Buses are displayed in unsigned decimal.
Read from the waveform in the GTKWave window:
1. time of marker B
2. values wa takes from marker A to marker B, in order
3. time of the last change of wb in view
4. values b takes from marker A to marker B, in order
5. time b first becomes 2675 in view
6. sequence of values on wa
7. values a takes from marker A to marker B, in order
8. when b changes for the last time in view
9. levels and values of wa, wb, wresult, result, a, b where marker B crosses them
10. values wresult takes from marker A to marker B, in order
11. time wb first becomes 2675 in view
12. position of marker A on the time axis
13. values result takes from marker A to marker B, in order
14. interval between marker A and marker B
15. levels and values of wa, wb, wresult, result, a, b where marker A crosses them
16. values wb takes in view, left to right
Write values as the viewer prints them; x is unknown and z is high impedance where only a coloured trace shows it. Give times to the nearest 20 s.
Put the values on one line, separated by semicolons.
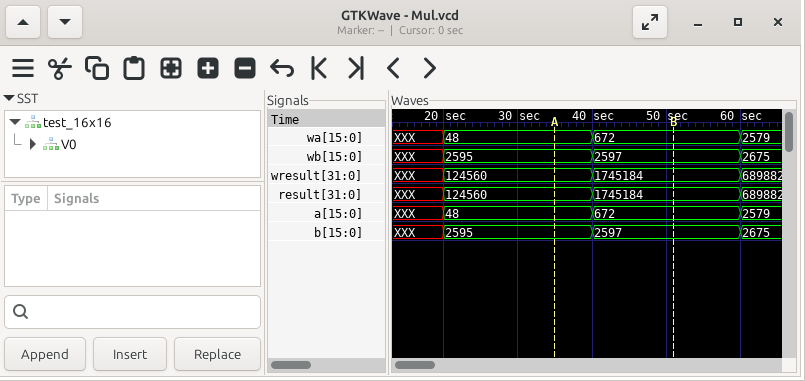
60 s; 48, 672; 60 s; 2595, 2597; 60 s; XXX, 48, 672, 2579; 48, 672; 60 s; wa=672, wb=2597, wresult=1745184, result=1745184, a=672, b=2597; 124560, 1745184; 60 s; 40 s; 124560, 1745184; 20 s; wa=48, wb=2595, wresult=124560, result=124560, a=48, b=2595; XXX, 2595, 2597, 2675
